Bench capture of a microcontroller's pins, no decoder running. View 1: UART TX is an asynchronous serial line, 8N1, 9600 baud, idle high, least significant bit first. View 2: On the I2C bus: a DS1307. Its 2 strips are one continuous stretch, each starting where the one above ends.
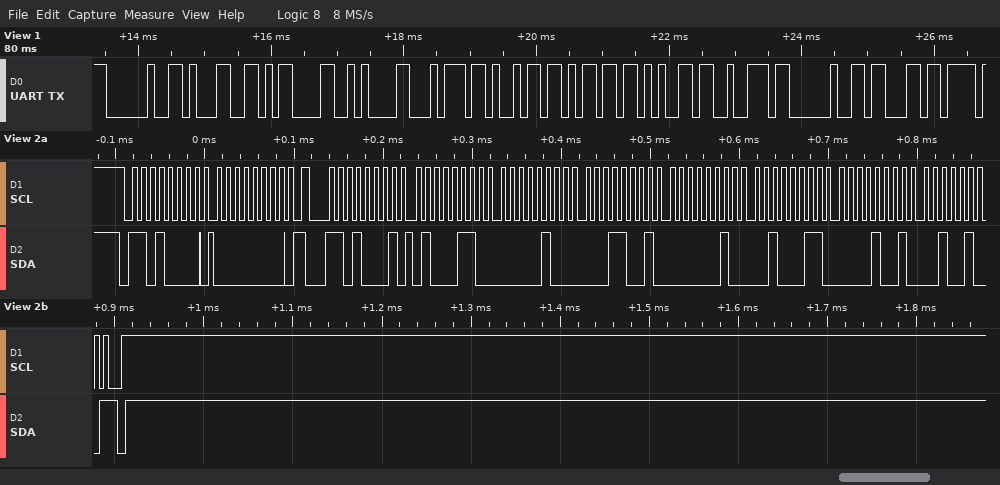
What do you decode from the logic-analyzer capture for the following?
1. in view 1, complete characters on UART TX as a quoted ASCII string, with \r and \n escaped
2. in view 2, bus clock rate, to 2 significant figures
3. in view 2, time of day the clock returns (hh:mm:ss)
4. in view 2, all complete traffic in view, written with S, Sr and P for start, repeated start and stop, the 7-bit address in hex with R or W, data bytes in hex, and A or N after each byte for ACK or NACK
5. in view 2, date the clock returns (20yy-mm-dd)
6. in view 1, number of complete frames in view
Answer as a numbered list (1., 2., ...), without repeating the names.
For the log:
1. " 1\r\ntimer c"
2. 100 kHz
3. 19:04:46
4. S 68W A 00 A Sr 68R A 46 A 04 A 19 A 02 A 23 A 09 A 24 N P
5. 2024-09-23
6. 11
